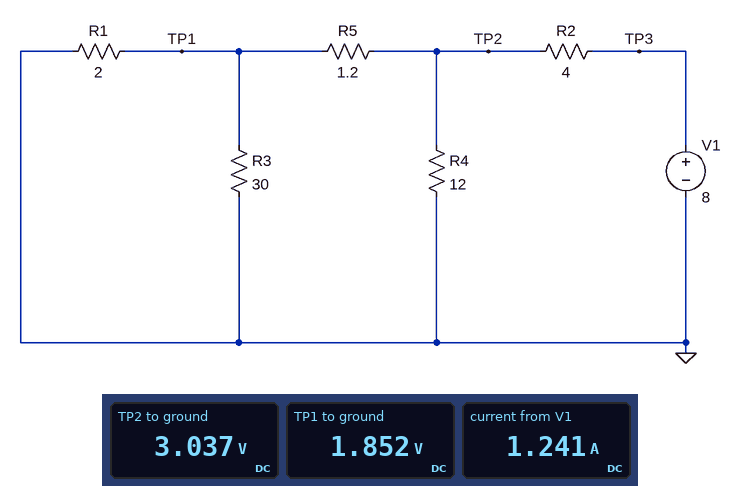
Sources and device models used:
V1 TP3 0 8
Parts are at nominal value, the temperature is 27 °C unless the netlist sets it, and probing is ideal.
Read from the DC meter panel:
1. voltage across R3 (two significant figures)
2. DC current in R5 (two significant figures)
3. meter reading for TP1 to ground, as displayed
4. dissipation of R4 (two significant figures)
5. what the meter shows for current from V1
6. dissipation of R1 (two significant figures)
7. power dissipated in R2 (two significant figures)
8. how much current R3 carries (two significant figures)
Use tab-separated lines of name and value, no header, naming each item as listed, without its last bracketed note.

voltage across R3	1.9 V
DC current in R5	990 mA
meter reading for TP1 to ground, as displayed	1.852 V
dissipation of R4	770 mW
what the meter shows for current from V1	1.241 A
dissipation of R1	1.7 W
power dissipated in R2	6.2 W
how much current R3 carries	62 mA
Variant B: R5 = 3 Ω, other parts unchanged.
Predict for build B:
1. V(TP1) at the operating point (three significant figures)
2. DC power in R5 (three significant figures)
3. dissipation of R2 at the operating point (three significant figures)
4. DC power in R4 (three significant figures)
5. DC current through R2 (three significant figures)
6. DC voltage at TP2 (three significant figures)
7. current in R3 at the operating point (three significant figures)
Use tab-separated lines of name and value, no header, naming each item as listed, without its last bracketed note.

V(TP1) at the operating point	1.43 V
DC power in R5	1.74 W
dissipation of R2 at the operating point	4.59 W
DC power in R4	1.15 W
DC current through R2	1.07 A
DC voltage at TP2	3.71 V
current in R3 at the operating point	47.6 mA
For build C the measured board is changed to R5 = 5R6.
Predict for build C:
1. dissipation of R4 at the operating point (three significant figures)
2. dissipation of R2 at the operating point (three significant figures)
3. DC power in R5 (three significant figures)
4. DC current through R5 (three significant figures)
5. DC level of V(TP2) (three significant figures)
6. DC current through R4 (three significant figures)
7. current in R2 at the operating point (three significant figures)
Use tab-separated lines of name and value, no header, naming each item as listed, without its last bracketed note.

dissipation of R4 at the operating point	1.53 W
dissipation of R2 at the operating point	3.46 W
DC power in R5	1.84 W
DC current through R5	573 mA
DC level of V(TP2)	4.28 V
DC current through R4	357 mA
current in R2 at the operating point	930 mA
